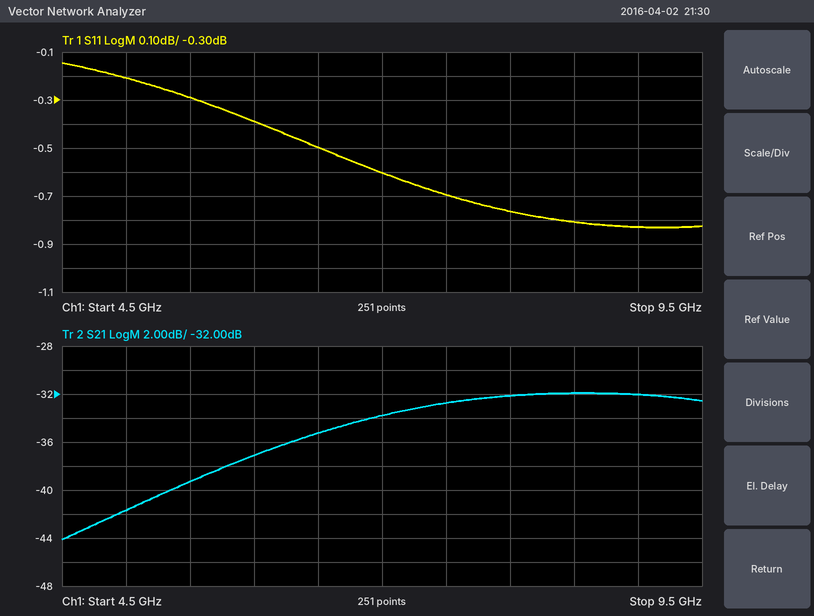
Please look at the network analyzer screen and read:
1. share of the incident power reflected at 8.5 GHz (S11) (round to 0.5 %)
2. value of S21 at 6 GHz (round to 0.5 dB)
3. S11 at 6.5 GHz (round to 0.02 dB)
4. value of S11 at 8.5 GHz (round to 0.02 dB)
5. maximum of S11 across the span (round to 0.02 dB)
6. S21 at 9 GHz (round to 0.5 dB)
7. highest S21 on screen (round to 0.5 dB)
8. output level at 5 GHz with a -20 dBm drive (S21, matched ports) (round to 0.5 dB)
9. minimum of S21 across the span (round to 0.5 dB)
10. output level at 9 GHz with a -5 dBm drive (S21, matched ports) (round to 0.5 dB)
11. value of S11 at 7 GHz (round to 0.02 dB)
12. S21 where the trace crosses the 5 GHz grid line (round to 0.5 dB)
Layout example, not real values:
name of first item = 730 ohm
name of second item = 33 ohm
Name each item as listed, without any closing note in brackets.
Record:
share of the incident power reflected at 8.5 GHz (S11) = 83.0 %
value of S21 at 6 GHz = -37.0 dB
S11 at 6.5 GHz = -0.50 dB
value of S11 at 8.5 GHz = -0.80 dB
maximum of S11 across the span = -0.14 dB
S21 at 9 GHz = -32.0 dB
highest S21 on screen = -32.0 dB
output level at 5 GHz with a -20 dBm drive (S21, matched ports) = -61.5 dBm
minimum of S21 across the span = -44.0 dB
output level at 9 GHz with a -5 dBm drive (S21, matched ports) = -37.0 dBm
value of S11 at 7 GHz = -0.60 dB
S21 where the trace crosses the 5 GHz grid line = -41.5 dB
